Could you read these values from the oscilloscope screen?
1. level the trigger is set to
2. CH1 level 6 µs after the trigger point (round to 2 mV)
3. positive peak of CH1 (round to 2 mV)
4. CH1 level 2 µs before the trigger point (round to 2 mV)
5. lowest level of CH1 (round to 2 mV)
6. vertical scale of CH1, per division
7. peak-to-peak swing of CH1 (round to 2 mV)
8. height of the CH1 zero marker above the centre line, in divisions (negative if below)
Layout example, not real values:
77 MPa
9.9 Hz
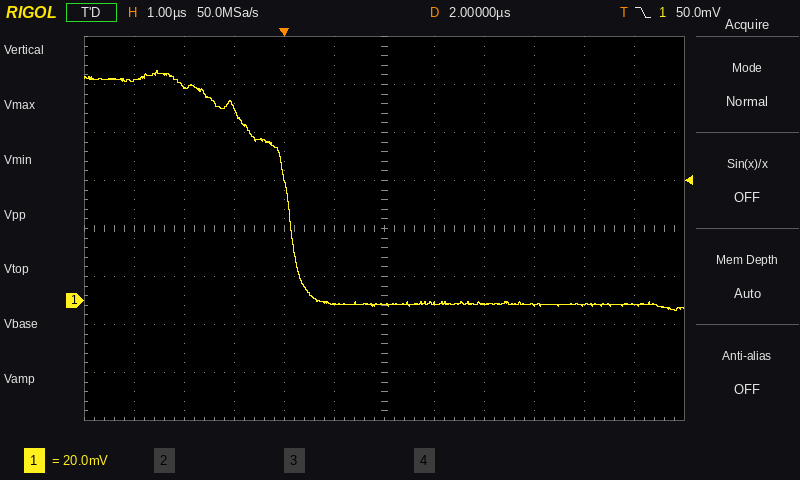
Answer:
50.0 mV
-2 mV
96 mV
90 mV
-4 mV
20 mV
100 mV
-1.5 div
